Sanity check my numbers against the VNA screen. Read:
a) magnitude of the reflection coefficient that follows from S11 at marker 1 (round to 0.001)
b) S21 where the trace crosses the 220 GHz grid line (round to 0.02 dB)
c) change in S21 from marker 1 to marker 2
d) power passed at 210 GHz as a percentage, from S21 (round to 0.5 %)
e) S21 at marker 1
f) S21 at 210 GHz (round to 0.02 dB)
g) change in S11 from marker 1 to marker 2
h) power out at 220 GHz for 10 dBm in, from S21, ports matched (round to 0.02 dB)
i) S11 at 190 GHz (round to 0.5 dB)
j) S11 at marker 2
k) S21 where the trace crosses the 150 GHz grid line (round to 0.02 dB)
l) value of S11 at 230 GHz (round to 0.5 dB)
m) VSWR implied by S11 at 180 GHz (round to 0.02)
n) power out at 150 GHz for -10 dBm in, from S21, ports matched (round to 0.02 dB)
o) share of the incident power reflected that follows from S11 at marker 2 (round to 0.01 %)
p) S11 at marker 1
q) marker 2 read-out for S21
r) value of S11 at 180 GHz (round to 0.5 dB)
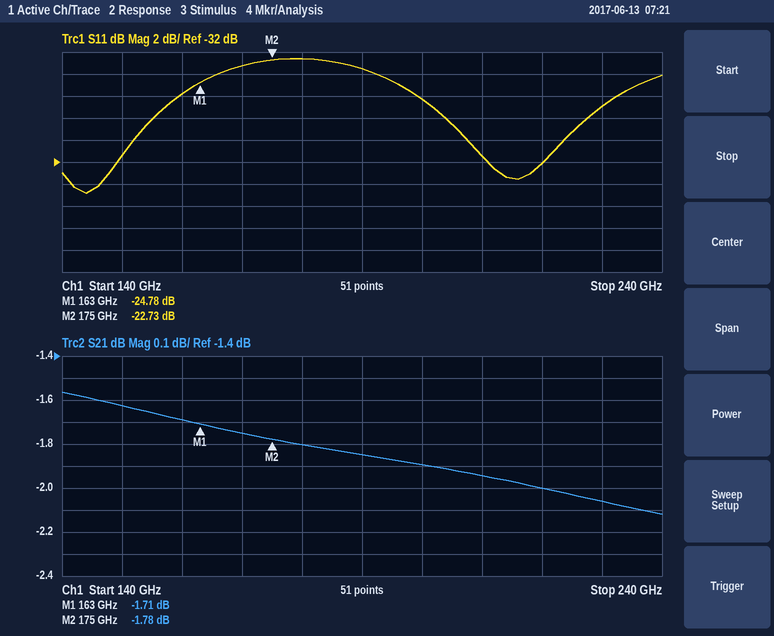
0.058
-2.00 dB
-0.07 dB
64.0 %
-1.71 dB
-1.94 dB
2.05 dB
8.00 dBm
-23.5 dB
-22.73 dB
-1.62 dB
-27.0 dB
1.16
-11.62 dBm
0.53 %
-24.78 dB
-1.78 dB
-22.5 dB
